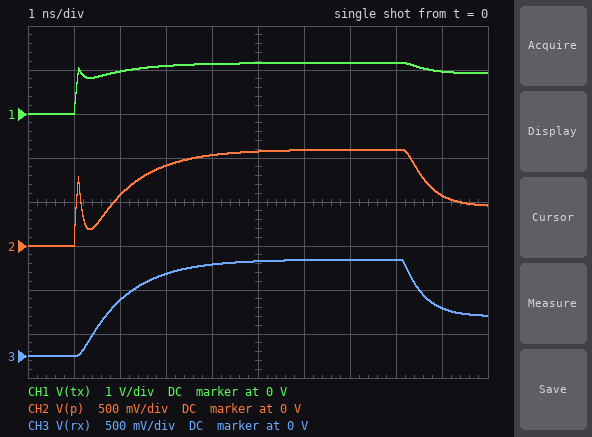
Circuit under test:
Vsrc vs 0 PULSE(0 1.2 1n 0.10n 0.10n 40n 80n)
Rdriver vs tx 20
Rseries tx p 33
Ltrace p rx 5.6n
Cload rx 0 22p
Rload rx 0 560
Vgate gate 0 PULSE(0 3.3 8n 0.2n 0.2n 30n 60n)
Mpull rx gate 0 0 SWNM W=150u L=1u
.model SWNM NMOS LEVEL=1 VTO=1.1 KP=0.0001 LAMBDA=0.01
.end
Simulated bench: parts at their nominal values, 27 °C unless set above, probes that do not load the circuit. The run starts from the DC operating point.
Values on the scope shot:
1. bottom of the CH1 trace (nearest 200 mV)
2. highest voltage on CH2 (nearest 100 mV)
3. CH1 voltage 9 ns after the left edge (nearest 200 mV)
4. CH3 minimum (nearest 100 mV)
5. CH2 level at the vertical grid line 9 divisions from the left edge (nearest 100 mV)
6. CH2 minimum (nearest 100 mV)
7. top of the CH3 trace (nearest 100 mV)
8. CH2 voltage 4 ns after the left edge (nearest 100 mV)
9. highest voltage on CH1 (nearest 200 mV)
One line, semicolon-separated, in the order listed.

0 V; 1.1 V; 1.0 V; 0 V; 600 mV; 0 V; 1.1 V; 1.0 V; 1.2 V
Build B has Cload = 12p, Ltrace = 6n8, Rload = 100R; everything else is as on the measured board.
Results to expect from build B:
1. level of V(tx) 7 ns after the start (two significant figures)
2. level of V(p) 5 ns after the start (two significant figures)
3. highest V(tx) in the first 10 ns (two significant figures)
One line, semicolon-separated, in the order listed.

1.0 V; 780 mV; 1.1 V
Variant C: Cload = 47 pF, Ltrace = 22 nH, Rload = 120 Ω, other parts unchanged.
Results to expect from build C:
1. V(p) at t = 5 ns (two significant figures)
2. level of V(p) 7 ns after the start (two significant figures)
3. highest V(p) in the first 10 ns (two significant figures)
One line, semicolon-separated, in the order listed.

730 mV; 810 mV; 1.1 V
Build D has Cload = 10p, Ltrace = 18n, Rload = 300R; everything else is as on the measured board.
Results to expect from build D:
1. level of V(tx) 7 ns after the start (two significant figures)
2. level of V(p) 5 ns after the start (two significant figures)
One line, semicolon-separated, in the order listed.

1.1 V; 1.0 V
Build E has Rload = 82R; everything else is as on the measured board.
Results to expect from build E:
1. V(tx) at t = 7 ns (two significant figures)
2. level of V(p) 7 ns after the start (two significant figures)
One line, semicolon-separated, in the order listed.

1.0 V; 730 mV
